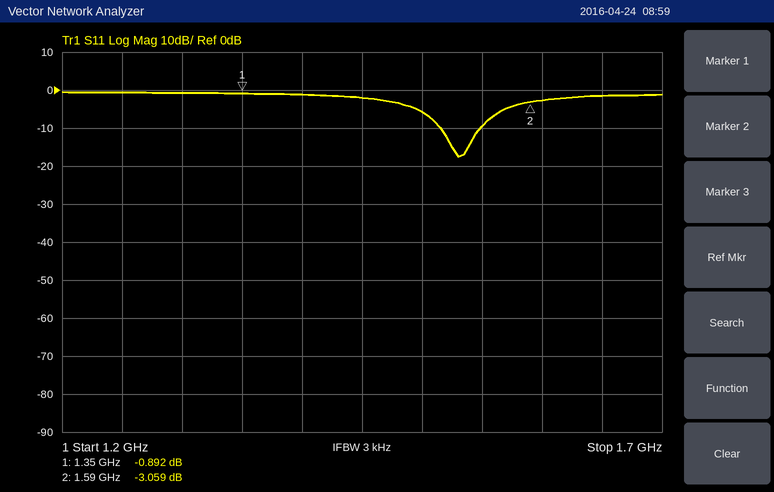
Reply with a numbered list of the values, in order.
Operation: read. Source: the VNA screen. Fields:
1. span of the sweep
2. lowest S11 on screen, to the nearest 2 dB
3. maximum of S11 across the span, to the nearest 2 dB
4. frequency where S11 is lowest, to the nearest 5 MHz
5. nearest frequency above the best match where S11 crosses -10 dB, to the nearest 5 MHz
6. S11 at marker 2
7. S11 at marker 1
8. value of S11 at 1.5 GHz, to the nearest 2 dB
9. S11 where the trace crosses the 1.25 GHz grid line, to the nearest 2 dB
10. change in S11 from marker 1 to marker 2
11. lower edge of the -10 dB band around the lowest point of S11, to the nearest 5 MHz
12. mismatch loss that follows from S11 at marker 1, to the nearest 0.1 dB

1. 500 MHz
2. -18 dB
3. 0 dB
4. 1.530 GHz
5. 1.550 GHz
6. -3.059 dB
7. -0.892 dB
8. -6 dB
9. 0 dB
10. -2.167 dB
11. 1.515 GHz
12. 7.3 dB
